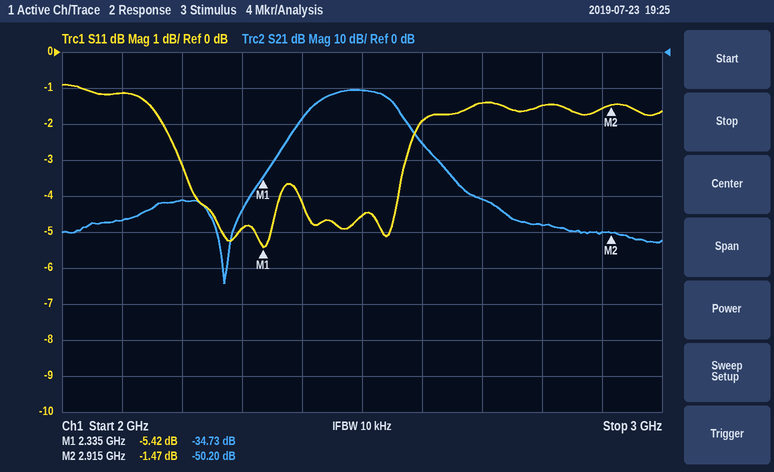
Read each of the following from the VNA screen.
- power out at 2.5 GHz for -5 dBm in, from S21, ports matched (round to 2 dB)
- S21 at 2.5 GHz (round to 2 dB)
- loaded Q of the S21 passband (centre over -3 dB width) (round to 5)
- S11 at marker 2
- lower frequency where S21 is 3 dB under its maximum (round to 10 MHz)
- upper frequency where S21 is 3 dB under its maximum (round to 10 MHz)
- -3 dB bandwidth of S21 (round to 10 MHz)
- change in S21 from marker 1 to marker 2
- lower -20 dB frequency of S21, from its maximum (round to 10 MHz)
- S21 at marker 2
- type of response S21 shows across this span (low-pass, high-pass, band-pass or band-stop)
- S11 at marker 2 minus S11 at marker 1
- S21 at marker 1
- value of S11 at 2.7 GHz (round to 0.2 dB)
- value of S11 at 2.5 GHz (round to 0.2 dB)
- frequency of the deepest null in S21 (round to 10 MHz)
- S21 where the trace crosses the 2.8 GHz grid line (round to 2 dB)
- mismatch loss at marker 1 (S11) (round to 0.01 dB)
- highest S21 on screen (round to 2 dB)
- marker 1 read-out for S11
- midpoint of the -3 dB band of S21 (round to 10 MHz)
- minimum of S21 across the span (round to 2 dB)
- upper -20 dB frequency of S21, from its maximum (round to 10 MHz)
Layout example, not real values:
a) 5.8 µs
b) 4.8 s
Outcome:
a) -16 dBm
b) -10 dB
c) 20
d) -1.47 dB
e) 2.43 GHz
f) 2.55 GHz
g) 120 MHz
h) -15.47 dB
i) 2.35 GHz
j) -50.20 dB
k) band-pass
l) 3.95 dB
m) -34.73 dB
n) -1.4 dB
o) -4.6 dB
p) 2.27 GHz
q) -48 dB
r) 1.47 dB
s) -10 dB
t) -5.42 dB
u) 2.49 GHz
v) -64 dB
w) 2.63 GHz
